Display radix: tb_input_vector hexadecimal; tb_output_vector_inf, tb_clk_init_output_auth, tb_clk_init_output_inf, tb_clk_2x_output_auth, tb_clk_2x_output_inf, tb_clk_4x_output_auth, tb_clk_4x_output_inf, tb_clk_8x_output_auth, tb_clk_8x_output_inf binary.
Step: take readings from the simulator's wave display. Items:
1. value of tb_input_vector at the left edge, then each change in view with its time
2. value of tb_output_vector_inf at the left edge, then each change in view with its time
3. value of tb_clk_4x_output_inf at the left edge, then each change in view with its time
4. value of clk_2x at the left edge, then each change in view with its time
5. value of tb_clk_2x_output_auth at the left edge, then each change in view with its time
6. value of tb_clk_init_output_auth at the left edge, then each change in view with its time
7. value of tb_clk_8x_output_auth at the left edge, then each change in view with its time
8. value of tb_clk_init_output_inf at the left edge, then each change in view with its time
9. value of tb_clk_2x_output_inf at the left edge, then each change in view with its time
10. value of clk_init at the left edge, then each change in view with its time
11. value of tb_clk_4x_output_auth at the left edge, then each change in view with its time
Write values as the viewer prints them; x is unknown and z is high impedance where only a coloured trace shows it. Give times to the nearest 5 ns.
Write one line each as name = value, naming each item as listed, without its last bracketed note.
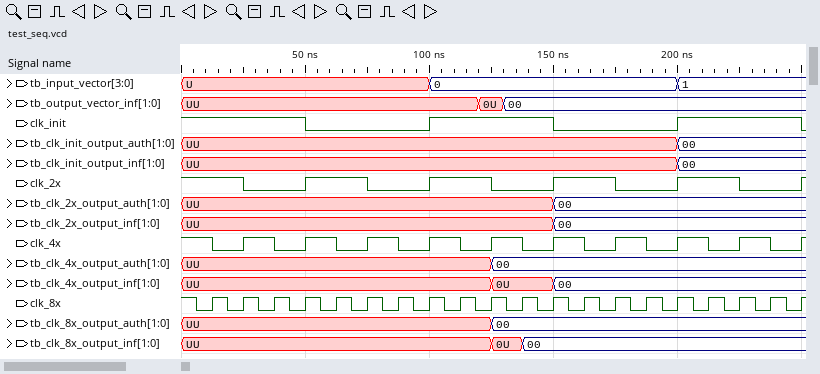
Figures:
value of tb_input_vector at the left edge, then each change in view with its time = U, 0 at 100 ns, 1 at 200 ns
value of tb_output_vector_inf at the left edge, then each change in view with its time = UU, 0U at 120 ns, 00 at 130 ns
value of tb_clk_4x_output_inf at the left edge, then each change in view with its time = UU, 0U at 125 ns, 00 at 150 ns
value of clk_2x at the left edge, then each change in view with its time = 1, 0 at 25 ns, 1 at 50 ns, 0 at 75 ns, 1 at 100 ns, 0 at 125 ns, 1 at 150 ns, 0 at 175 ns, 1 at 200 ns, 0 at 225 ns, 1 at 250 ns
value of tb_clk_2x_output_auth at the left edge, then each change in view with its time = UU, 00 at 150 ns
value of tb_clk_init_output_auth at the left edge, then each change in view with its time = UU, 00 at 200 ns
value of tb_clk_8x_output_auth at the left edge, then each change in view with its time = UU, 00 at 125 ns
value of tb_clk_init_output_inf at the left edge, then each change in view with its time = UU, 00 at 200 ns
value of tb_clk_2x_output_inf at the left edge, then each change in view with its time = UU, 00 at 150 ns
value of clk_init at the left edge, then each change in view with its time = 1, 0 at 50 ns, 1 at 100 ns, 0 at 150 ns, 1 at 200 ns, 0 at 250 ns
value of tb_clk_4x_output_auth at the left edge, then each change in view with its time = UU, 00 at 125 ns
